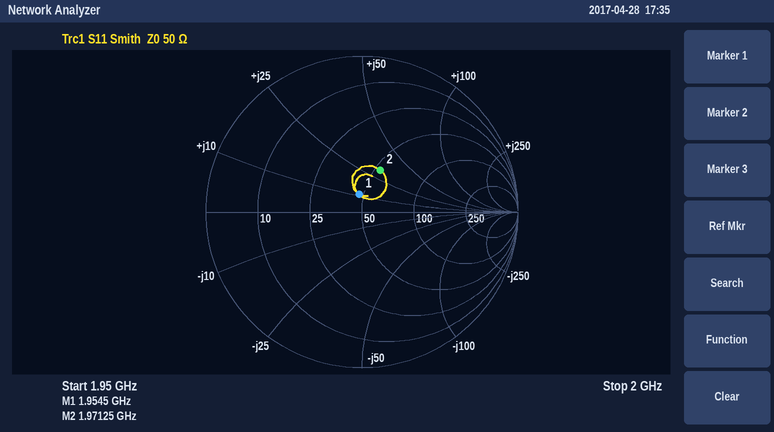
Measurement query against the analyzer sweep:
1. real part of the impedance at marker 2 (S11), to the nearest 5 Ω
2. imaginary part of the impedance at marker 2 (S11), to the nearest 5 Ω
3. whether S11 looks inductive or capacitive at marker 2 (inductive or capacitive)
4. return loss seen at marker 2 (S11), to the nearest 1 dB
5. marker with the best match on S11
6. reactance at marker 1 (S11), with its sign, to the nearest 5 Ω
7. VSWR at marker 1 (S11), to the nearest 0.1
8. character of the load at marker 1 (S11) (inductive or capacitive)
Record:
55 Ω
+30 Ω
inductive
11 dB
marker 1
+10 Ω
1.3
inductive
